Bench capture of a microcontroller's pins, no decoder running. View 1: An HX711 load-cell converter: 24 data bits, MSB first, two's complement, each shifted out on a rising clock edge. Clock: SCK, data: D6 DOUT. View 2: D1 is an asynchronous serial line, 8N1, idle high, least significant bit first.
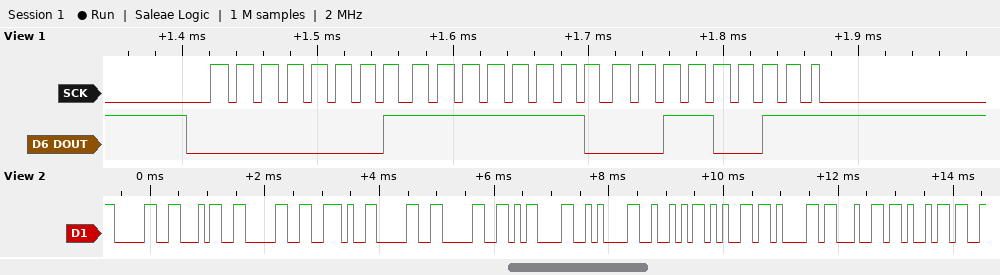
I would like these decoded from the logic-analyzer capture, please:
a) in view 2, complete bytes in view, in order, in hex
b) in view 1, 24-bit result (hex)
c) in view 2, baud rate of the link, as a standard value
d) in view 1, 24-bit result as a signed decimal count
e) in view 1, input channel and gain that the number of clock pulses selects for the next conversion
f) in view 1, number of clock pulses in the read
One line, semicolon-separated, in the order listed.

30 34 30 2E 30 30 0D 0A 52 65 61 64 69; 0x01FE33; 9600 baud; 130611; channel A, gain 128; 25
